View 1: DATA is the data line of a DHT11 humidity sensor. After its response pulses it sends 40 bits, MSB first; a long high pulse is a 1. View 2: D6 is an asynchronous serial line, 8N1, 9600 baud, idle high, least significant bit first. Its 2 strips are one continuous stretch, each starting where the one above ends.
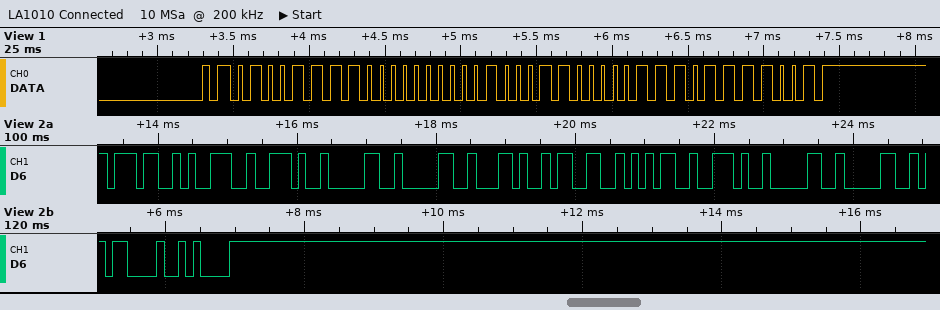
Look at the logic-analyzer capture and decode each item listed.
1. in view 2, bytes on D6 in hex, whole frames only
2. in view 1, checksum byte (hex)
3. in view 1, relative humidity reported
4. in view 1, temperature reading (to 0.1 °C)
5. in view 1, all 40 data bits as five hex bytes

37 39 2E 30 30 2C 33 35 2E 30 30 0D 0A
0x79
79 %
35.7 °C
4F 00 23 07 79
